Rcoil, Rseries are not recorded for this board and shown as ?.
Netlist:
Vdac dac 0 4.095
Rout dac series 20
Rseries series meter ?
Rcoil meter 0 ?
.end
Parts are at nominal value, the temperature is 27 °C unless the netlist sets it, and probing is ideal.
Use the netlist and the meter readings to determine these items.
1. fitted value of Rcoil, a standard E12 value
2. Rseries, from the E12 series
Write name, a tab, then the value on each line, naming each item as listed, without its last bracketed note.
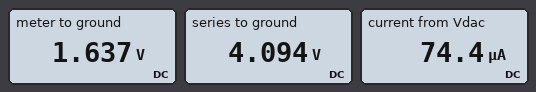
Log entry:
fitted value of Rcoil, a standard E12 value	22 kΩ
Rseries, from the E12 series	33 kΩ
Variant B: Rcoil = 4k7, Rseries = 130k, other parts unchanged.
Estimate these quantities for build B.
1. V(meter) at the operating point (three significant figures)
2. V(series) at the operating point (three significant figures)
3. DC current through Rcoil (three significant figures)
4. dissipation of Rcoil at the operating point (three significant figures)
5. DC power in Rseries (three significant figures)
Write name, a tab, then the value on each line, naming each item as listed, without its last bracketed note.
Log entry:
V(meter) at the operating point	143 mV
V(series) at the operating point	4.09 V
DC current through Rcoil	30.4 µA
dissipation of Rcoil at the operating point	4.34 µW
DC power in Rseries	120 µW
